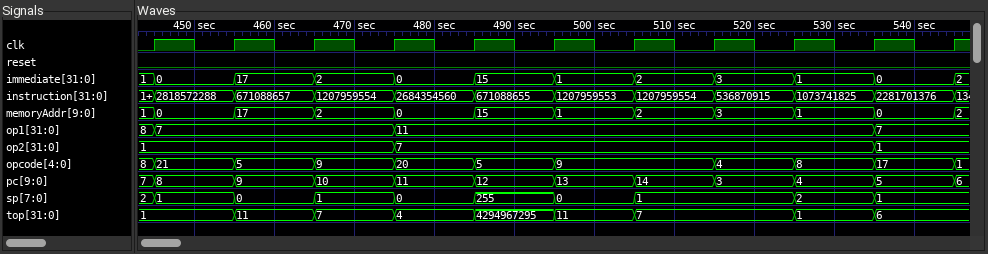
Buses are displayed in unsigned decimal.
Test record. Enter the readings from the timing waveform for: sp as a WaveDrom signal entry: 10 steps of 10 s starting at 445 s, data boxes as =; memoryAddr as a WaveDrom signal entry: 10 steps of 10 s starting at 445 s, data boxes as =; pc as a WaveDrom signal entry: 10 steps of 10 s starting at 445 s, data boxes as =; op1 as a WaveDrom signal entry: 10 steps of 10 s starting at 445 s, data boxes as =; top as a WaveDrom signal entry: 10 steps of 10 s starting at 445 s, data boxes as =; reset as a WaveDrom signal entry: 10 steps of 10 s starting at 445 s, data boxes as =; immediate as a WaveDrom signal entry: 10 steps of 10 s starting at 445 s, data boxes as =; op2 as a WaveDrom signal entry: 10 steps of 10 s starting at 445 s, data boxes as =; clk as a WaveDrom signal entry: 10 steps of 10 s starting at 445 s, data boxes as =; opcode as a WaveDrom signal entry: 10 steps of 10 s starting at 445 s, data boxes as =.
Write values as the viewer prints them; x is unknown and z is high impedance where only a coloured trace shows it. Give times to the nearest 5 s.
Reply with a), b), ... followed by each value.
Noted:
a) {name: 'sp', wave: '=======.==', data: '1 0 1 0 255 0 1 2 1'}
b) {name: 'memoryAddr', wave: '==========', data: '0 17 2 0 15 1 2 3 1 0'}
c) {name: 'pc', wave: '==========', data: '8 9 10 11 12 13 14 3 4 5'}
d) {name: 'op1', wave: '=..=.....=', data: '7 11 7'}
e) {name: 'top', wave: '=======.==', data: '1 11 7 4 4294967295 11 7 1 6'}
f) {name: 'reset', wave: '0.........'}
g) {name: 'immediate', wave: '==========', data: '0 17 2 0 15 1 2 3 1 0'}
h) {name: 'op2', wave: '=..=.....=', data: '1 7 1'}
i) {name: 'clk', wave: 'p.........'}
j) {name: 'opcode', wave: '======.===', data: '21 5 9 20 5 9 4 8 17'}
